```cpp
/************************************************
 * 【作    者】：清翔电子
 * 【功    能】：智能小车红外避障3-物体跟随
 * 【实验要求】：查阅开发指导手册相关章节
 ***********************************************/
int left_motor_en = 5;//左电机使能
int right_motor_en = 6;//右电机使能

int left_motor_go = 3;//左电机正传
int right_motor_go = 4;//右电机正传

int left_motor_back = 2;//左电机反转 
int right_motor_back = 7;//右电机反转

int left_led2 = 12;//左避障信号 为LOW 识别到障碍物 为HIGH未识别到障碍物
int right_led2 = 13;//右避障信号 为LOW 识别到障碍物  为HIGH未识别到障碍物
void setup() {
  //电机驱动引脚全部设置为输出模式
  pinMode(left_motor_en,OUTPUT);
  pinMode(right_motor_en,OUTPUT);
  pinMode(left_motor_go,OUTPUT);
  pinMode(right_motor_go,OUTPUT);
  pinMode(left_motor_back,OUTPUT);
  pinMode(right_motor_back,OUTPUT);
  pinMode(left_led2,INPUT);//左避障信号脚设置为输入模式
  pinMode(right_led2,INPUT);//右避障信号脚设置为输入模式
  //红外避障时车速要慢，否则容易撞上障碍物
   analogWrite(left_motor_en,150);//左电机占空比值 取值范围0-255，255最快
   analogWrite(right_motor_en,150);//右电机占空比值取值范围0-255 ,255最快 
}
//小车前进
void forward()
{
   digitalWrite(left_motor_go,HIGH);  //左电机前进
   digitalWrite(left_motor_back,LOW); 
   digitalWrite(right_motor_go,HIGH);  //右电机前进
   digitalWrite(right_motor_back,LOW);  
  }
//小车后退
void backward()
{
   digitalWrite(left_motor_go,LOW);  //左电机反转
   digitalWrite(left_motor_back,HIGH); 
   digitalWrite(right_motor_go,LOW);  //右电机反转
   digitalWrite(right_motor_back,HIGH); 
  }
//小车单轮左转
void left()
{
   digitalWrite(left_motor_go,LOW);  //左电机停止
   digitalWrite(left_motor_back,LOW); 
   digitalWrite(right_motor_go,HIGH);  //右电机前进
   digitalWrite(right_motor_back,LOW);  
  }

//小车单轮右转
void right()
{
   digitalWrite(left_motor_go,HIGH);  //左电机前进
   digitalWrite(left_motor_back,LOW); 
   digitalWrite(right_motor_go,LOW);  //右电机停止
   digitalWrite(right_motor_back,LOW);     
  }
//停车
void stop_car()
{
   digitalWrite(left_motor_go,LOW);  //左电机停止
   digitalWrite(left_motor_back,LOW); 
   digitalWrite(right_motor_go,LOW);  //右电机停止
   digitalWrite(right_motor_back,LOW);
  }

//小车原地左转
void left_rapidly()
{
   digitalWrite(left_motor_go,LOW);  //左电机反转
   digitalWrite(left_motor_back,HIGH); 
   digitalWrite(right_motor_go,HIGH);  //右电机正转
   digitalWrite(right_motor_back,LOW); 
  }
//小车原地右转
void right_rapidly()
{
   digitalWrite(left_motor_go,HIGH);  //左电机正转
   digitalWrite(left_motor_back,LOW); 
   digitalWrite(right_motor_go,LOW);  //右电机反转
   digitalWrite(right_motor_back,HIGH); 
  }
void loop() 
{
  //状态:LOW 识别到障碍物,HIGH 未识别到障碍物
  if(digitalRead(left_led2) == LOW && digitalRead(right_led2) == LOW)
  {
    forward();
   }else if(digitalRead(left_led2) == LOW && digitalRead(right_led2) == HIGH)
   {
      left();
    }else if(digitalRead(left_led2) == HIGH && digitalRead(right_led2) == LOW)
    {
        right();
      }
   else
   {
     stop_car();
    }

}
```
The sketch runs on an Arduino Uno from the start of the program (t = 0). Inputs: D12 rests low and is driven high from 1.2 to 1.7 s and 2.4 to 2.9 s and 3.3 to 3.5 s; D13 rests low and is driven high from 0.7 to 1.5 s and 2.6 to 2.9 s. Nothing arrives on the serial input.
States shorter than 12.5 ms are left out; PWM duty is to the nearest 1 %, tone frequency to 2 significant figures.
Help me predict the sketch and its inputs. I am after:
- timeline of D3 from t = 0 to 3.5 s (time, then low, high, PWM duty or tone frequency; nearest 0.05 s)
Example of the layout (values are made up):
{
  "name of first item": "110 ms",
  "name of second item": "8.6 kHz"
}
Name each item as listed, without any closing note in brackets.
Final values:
{
  "timeline of D3 from t = 0 to 3.5 s": "0 s high; 0.7 s low; 1.5 s high; 2.6 s low; 2.9 s high"
}
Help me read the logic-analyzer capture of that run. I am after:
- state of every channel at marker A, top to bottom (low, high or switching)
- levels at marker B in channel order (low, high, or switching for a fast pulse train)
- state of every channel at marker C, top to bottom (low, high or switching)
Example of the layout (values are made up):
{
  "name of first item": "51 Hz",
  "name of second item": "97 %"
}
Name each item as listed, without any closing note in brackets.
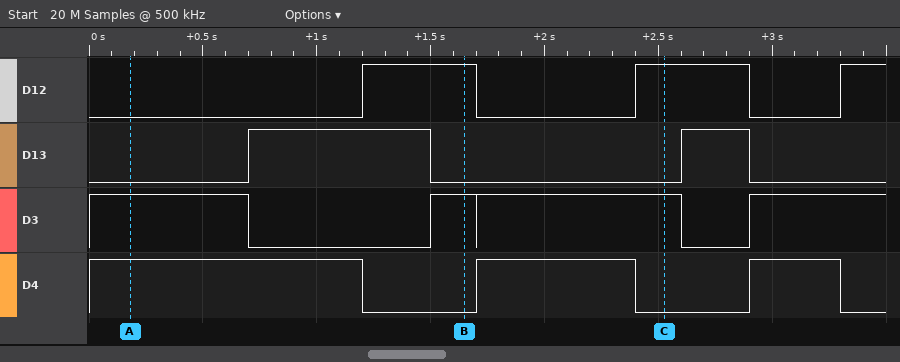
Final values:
{
  "state of every channel at marker A, top to bottom": "D12 low, D13 low, D3 high, D4 high",
  "levels at marker B in channel order": "D12 high, D13 low, D3 high, D4 low",
  "state of every channel at marker C, top to bottom": "D12 high, D13 low, D3 high, D4 low"
}
